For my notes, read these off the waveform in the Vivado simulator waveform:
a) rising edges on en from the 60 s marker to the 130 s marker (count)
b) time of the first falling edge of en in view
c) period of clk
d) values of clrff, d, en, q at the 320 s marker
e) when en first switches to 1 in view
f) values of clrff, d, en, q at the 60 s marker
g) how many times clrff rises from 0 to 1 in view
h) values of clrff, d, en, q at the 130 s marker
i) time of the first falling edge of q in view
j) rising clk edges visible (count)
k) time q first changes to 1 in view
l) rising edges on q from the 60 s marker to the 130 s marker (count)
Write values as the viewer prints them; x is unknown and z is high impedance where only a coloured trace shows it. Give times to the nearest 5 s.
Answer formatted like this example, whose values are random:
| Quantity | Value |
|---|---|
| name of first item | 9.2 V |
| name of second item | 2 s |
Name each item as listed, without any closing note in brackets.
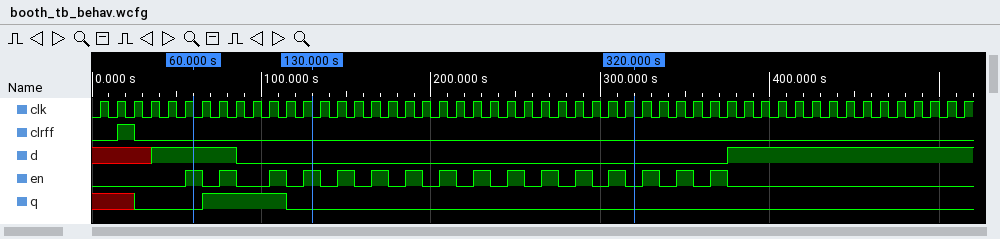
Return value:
| Quantity | Value |
|---|---|
| rising edges on en from the 60 s marker to the 130 s marker | 3 |
| time of the first falling edge of en in view | 65 s |
| period of clk | 10 s |
| values of clrff, d, en, q at the 320 s marker | clrff=0, d=0, en=0, q=0 |
| when en first switches to 1 in view | 55 s |
| values of clrff, d, en, q at the 60 s marker | clrff=0, d=1, en=1, q=0 |
| how many times clrff rises from 0 to 1 in view | 1 |
| values of clrff, d, en, q at the 130 s marker | clrff=0, d=0, en=1, q=0 |
| time of the first falling edge of q in view | 115 s |
| rising clk edges visible | 52 |
| time q first changes to 1 in view | 65 s |
| rising edges on q from the 60 s marker to the 130 s marker | 1 |
